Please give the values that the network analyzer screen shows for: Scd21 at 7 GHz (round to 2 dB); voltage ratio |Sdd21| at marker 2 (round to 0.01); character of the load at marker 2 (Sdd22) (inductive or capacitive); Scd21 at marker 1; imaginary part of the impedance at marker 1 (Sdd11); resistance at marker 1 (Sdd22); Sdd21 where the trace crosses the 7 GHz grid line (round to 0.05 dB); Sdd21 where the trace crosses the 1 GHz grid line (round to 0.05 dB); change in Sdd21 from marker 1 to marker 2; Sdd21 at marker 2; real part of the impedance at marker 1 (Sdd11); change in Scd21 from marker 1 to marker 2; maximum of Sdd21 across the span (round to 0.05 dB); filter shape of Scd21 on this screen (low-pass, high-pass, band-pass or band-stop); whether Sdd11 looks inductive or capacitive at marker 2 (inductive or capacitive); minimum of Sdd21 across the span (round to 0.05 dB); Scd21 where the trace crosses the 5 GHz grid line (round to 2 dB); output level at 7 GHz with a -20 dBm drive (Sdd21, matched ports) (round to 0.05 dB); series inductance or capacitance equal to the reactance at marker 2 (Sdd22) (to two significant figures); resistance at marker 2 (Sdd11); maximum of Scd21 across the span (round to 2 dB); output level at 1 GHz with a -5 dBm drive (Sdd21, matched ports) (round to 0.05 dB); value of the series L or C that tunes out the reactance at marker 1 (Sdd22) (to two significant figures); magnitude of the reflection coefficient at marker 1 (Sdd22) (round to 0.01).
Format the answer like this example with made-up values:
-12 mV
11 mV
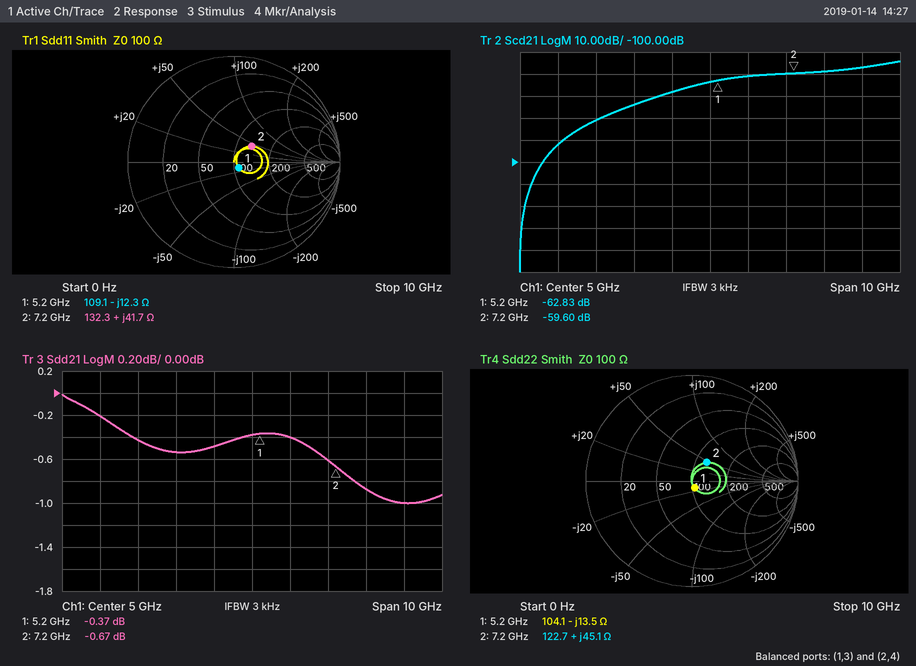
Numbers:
-60 dB
0.93
inductive
-62.83 dB
-12.3 Ω
104.1 Ω
-0.60 dB
-0.20 dB
-0.30 dB
-0.67 dB
109.1 Ω
3.23 dB
0.00 dB
high-pass
inductive
-1.00 dB
-64 dB
-20.60 dBm
1.00 nH
132.3 Ω
-54 dB
-5.20 dBm
410 pH
0.07
